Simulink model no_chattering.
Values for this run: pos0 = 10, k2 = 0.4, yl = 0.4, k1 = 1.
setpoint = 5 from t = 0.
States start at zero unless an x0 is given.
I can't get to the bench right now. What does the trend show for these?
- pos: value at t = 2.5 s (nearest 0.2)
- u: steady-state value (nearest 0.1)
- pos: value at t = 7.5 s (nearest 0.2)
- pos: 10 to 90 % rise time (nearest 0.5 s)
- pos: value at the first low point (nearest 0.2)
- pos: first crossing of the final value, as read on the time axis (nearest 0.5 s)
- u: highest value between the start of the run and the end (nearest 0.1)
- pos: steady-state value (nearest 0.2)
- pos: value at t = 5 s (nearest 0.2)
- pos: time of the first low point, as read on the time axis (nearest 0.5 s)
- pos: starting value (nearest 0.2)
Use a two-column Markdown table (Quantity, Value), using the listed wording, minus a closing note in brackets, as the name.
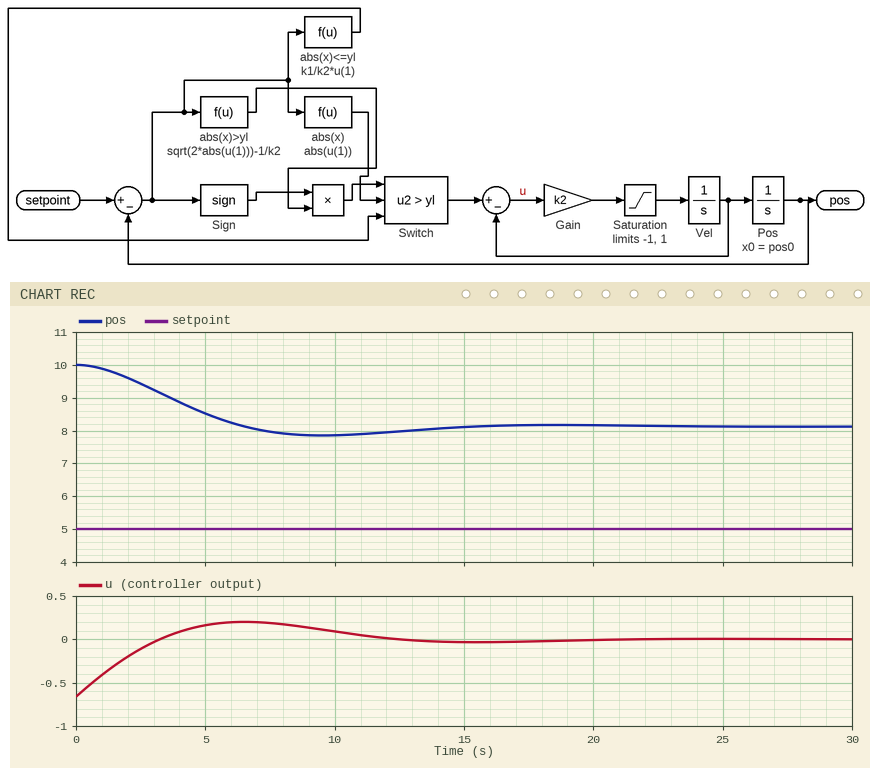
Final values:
| Quantity | Value |
|---|---|
| pos: value at t = 2.5 s | 9.4 |
| u: steady-state value | 0.0 |
| pos: value at t = 7.5 s | 8.0 |
| pos: 10 to 90 % rise time | 4.5 s |
| pos: value at the first low point | 7.8 |
| pos: first crossing of the final value, as read on the time axis | 6.5 s |
| u: highest value between the start of the run and the end | 0.2 |
| pos: steady-state value | 8.2 |
| pos: value at t = 5 s | 8.6 |
| pos: time of the first low point, as read on the time axis | 9.5 s |
| pos: starting value | 10.0 |
